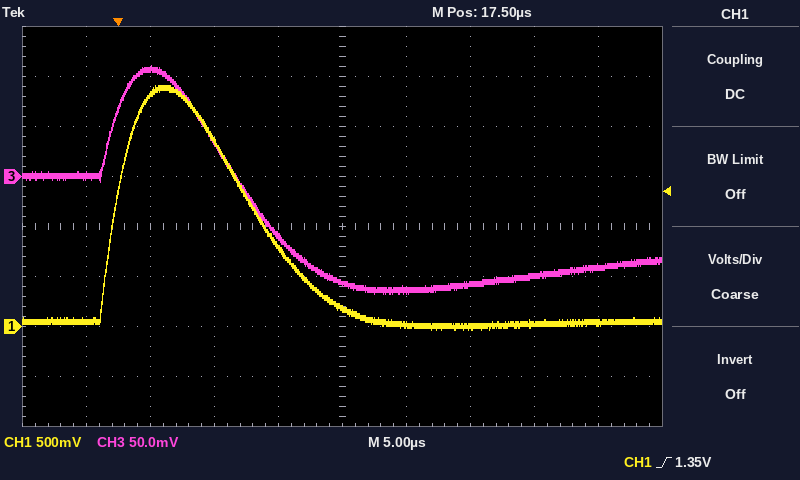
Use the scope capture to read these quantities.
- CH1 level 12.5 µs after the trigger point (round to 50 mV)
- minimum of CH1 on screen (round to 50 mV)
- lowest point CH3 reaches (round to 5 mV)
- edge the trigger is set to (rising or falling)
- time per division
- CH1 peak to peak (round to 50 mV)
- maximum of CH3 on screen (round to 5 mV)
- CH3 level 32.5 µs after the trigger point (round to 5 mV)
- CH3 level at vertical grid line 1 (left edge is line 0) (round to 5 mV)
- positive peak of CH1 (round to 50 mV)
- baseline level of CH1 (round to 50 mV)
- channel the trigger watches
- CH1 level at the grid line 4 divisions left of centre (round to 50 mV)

800 mV
-50 mV
-115 mV
rising
5 µs
2.45 V
110 mV
-100 mV
0 mV
2.40 V
50 mV
CH1
50 mV
